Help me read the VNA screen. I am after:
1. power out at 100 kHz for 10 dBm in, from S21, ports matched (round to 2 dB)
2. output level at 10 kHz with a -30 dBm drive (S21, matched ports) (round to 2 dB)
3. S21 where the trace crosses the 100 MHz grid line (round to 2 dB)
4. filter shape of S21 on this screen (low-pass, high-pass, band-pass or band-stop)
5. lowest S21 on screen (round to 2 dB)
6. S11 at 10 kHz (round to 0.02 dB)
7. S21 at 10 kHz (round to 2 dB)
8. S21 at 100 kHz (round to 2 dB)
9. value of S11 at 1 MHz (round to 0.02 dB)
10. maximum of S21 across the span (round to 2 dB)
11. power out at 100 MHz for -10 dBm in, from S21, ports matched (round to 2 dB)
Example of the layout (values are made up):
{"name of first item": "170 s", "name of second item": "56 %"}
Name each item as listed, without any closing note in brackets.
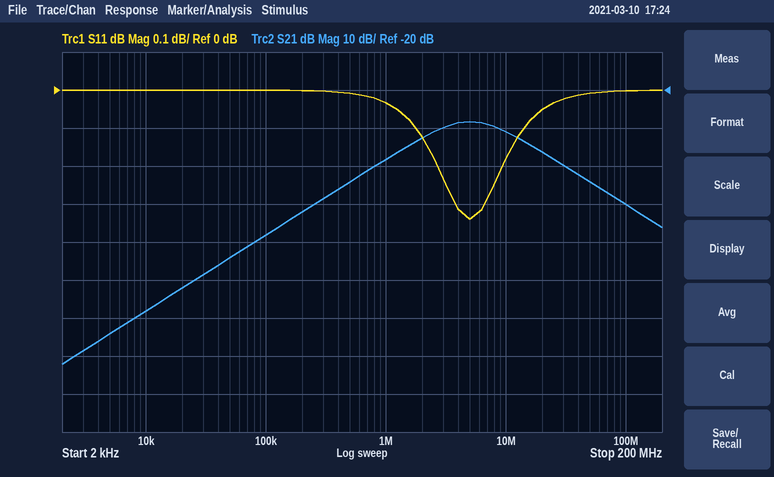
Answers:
{"power out at 100 kHz for 10 dBm in, from S21, ports matched": "-48 dBm", "output level at 10 kHz with a -30 dBm drive (S21, matched ports)": "-108 dBm", "S21 where the trace crosses the 100 MHz grid line": "-50 dB", "filter shape of S21 on this screen": "band-pass", "lowest S21 on screen": "-92 dB", "S11 at 10 kHz": "0.00 dB", "S21 at 10 kHz": "-78 dB", "S21 at 100 kHz": "-58 dB", "value of S11 at 1 MHz": "-0.04 dB", "maximum of S21 across the span": "-28 dB", "power out at 100 MHz for -10 dBm in, from S21, ports matched": "-60 dBm"}
